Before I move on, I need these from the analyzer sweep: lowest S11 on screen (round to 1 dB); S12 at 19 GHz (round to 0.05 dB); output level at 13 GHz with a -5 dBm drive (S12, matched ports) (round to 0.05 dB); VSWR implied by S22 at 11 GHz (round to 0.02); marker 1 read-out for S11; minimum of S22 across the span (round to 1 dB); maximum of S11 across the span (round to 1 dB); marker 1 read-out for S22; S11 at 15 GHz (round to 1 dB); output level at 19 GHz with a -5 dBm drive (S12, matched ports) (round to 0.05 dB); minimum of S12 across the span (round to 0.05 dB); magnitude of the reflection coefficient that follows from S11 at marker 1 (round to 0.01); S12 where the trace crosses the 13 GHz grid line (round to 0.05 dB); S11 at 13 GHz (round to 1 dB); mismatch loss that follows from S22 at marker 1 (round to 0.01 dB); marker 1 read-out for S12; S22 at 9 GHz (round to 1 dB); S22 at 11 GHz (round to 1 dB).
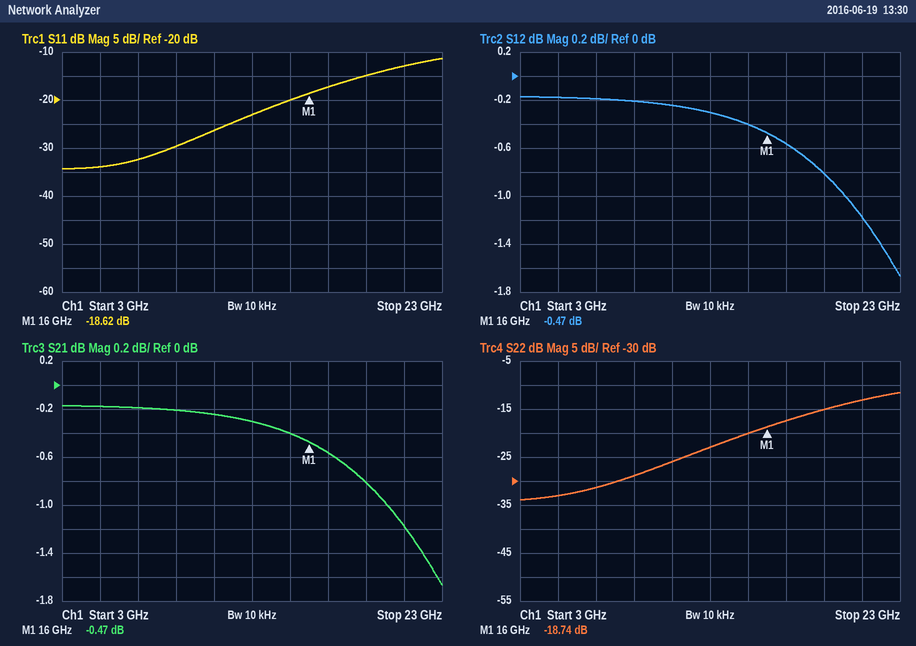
-34 dB
-0.80 dB
-5.30 dBm
1.10
-18.62 dB
-34 dB
-11 dB
-18.74 dB
-20 dB
-5.80 dBm
-1.65 dB
0.12
-0.30 dB
-23 dB
0.06 dB
-0.47 dB
-29 dB
-26 dB
